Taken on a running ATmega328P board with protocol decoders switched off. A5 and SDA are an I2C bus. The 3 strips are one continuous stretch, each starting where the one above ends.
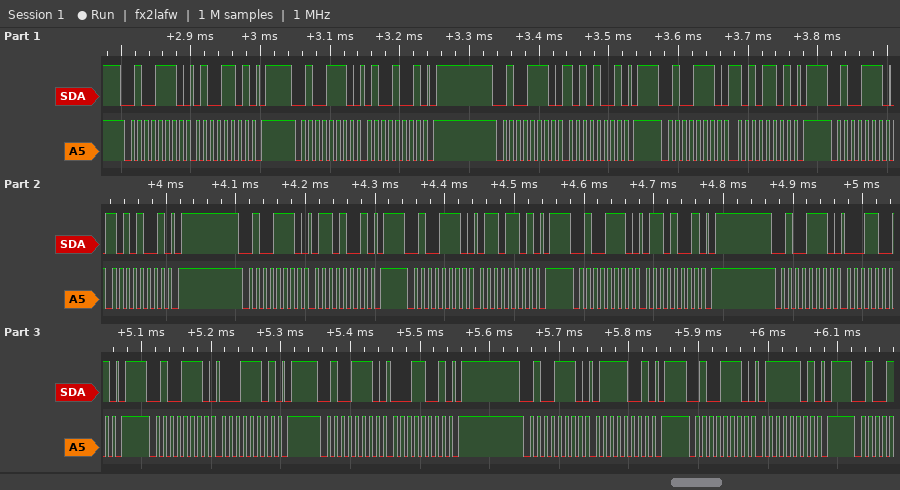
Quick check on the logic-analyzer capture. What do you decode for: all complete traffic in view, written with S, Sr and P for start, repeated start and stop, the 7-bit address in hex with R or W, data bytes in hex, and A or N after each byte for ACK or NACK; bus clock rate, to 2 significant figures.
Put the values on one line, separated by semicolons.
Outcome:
S 27W A 4D A P S 27W A 49 A P S 27W A A9 A P S 27W A AD A P S 27W A A9 A P S 27W A 69 A P S 27W A 6D A P S 27W A 69 A P S 27W A 19 A P S 27W A 1D A P S 27W A 19 A P S 27W A 79 A P S 27W A 7D A P; 100 kHz
